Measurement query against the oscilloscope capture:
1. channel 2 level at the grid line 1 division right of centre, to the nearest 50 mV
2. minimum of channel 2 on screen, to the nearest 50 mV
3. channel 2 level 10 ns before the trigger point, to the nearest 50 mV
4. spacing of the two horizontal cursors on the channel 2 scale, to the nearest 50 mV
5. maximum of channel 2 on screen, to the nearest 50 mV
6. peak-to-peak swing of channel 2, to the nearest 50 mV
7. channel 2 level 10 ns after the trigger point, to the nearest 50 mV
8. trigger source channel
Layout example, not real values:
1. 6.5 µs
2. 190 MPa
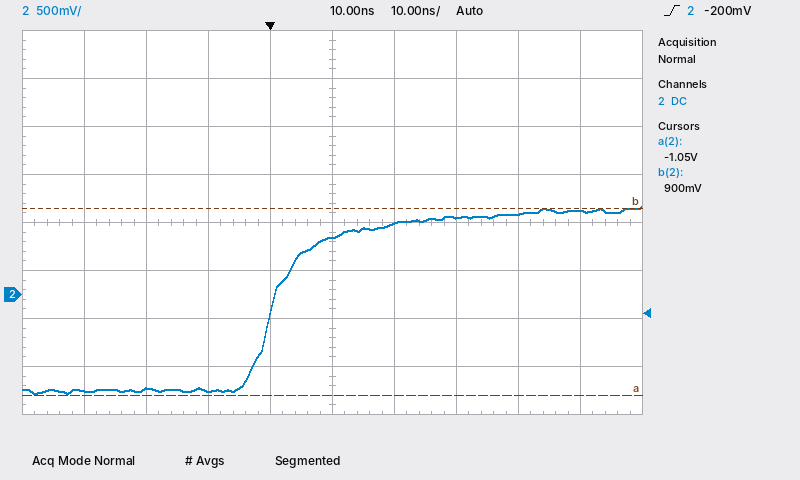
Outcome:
1. 750 mV
2. -1.05 V
3. -1.00 V
4. 1.95 V
5. 900 mV
6. 1.95 V
7. 600 mV
8. channel 2
